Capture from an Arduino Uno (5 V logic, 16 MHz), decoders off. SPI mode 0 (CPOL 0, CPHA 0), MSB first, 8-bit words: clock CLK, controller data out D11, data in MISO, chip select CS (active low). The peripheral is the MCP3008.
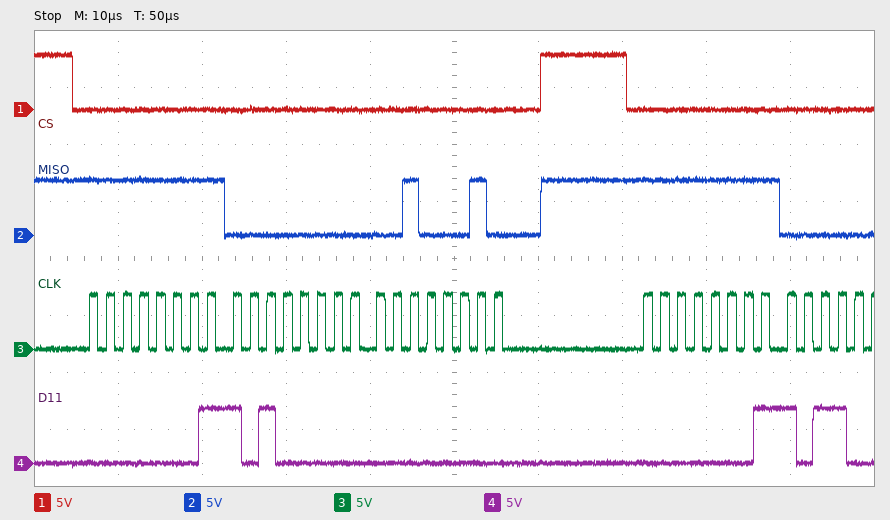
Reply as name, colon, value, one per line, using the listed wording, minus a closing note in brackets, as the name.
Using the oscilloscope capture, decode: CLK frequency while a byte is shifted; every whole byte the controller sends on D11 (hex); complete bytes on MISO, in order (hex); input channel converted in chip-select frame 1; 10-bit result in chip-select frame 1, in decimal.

CLK frequency while a byte is shifted: 500 kHz
every whole byte the controller sends on D11: 01 A0 00 01
complete bytes on MISO, in order: FF 00 22 FF
input channel converted in chip-select frame 1: 2
10-bit result in chip-select frame 1, in decimal: 34
